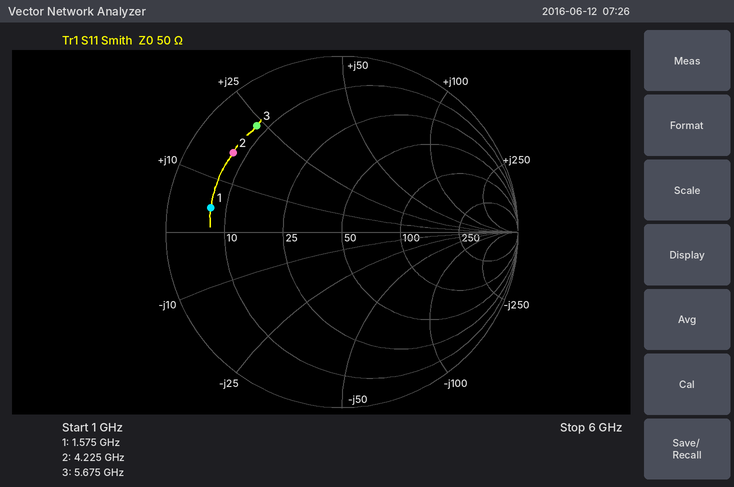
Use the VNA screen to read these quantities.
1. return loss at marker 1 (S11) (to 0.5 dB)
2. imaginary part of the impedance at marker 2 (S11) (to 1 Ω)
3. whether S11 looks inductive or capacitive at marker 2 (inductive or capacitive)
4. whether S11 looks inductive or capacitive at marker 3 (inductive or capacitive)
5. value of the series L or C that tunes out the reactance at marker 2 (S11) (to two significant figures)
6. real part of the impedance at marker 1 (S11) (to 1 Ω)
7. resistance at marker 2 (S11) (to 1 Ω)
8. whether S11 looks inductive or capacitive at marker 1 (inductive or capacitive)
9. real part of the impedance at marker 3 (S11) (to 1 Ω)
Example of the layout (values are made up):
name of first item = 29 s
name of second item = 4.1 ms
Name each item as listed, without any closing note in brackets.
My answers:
return loss at marker 1 (S11) = 2.5 dB
imaginary part of the impedance at marker 2 (S11) = +16 Ω
whether S11 looks inductive or capacitive at marker 2 = inductive
whether S11 looks inductive or capacitive at marker 3 = inductive
value of the series L or C that tunes out the reactance at marker 2 (S11) = 2.4 pF
real part of the impedance at marker 1 (S11) = 7 Ω
resistance at marker 2 (S11) = 7 Ω
whether S11 looks inductive or capacitive at marker 1 = inductive
real part of the impedance at marker 3 (S11) = 8 Ω
